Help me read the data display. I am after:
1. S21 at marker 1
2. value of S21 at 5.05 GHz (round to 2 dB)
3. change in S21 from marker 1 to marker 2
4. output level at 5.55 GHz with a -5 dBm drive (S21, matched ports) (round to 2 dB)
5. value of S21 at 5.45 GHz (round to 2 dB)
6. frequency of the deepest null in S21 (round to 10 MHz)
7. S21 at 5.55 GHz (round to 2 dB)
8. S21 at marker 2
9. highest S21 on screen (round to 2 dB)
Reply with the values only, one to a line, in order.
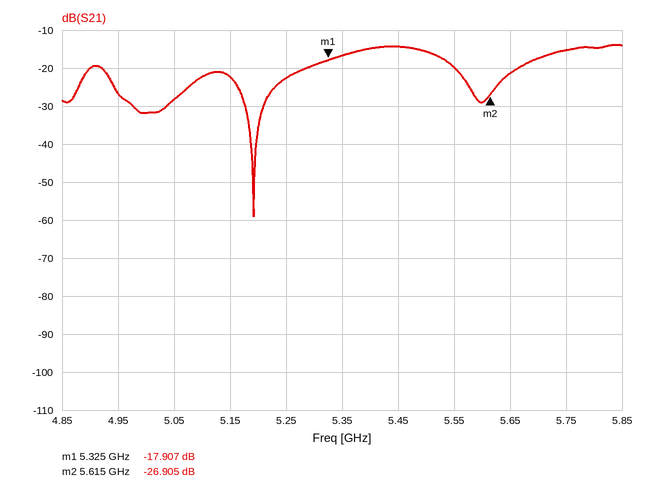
-17.907 dB
-28 dB
-8.998 dB
-24 dBm
-14 dB
5.19 GHz
-20 dB
-26.905 dB
-14 dB
